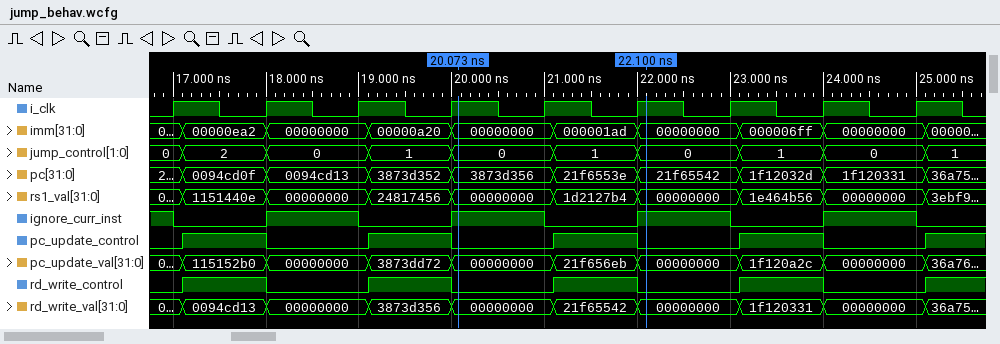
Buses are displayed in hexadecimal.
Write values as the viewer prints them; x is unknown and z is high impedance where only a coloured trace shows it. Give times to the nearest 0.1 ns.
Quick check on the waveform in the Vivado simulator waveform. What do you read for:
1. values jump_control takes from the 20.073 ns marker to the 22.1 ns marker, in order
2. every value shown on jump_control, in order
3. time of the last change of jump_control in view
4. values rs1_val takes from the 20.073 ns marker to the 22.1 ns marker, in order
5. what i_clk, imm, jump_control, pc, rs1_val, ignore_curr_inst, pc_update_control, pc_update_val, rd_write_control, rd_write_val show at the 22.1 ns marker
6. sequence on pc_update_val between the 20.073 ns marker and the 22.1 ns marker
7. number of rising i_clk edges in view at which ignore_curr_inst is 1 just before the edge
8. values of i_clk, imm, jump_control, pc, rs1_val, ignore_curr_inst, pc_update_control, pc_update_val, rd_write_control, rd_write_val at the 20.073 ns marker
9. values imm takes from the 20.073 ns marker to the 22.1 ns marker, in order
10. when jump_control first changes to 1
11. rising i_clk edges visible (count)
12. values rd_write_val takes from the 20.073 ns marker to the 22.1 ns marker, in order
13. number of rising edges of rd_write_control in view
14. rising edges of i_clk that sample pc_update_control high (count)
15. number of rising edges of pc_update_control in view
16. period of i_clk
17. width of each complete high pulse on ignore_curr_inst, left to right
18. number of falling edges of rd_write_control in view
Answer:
0, 1, 0
0, 2, 0, 1, 0, 1, 0, 1, 0, 1
25.1 ns
00000000, 1d2127b4, 00000000
i_clk=1, imm=00000000, jump_control=0, pc=21f65542, rs1_val=00000000, ignore_curr_inst=1, pc_update_control=0, pc_update_val=00000000, rd_write_control=0, rd_write_val=00000000
00000000, 21f656eb, 00000000
5
i_clk=1, imm=00000000, jump_control=0, pc=3873d356, rs1_val=00000000, ignore_curr_inst=1, pc_update_control=0, pc_update_val=00000000, rd_write_control=0, rd_write_val=00000000
00000000, 000001ad, 00000000
19.1 ns
9
00000000, 21f65542, 00000000
5
4
5
1 ns
1 ns, 1 ns, 1 ns, 1 ns
4
